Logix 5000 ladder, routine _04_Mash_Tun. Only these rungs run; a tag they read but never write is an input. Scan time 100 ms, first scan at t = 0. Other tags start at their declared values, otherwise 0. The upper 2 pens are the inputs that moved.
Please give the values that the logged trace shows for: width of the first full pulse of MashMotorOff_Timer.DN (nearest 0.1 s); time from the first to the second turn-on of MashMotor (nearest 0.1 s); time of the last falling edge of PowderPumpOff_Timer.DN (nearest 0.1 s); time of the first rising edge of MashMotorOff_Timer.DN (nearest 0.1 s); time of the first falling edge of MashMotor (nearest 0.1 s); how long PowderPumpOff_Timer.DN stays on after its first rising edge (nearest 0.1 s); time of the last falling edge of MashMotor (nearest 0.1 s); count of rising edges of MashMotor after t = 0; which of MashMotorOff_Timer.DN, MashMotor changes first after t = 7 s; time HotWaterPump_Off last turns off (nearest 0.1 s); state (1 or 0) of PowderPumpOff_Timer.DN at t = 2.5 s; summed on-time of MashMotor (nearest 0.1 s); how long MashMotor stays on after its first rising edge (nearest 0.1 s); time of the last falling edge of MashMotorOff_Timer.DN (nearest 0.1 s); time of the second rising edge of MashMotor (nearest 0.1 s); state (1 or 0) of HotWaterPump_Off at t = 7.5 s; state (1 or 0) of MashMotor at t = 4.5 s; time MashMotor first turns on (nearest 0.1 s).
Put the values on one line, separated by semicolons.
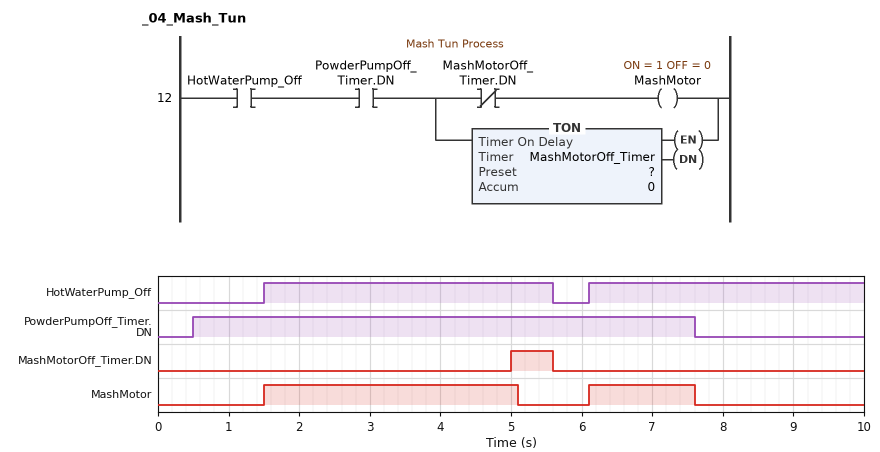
0.6 s; 4.6 s; 7.6 s; 5.0 s; 5.1 s; 7.1 s; 7.6 s; 2; MashMotor; 5.6 s; 1; 5.1 s; 3.6 s; 5.6 s; 6.1 s; 1; 1; 1.5 s
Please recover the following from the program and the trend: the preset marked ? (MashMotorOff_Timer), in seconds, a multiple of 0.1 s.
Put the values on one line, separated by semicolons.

3.5 s
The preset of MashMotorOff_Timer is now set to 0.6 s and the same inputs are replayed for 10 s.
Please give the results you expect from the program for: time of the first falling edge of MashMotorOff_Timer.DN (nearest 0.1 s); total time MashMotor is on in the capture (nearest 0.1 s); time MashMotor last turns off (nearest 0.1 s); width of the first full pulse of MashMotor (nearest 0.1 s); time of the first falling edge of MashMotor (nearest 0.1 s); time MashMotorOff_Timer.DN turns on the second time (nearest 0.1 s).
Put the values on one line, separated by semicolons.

5.6 s; 1.4 s; 6.8 s; 0.7 s; 2.2 s; 6.7 s
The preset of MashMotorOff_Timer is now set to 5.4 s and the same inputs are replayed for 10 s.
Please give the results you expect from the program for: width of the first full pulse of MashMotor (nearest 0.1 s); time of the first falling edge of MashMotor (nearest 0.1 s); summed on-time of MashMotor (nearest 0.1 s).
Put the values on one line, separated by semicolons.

4.1 s; 5.6 s; 5.6 s
